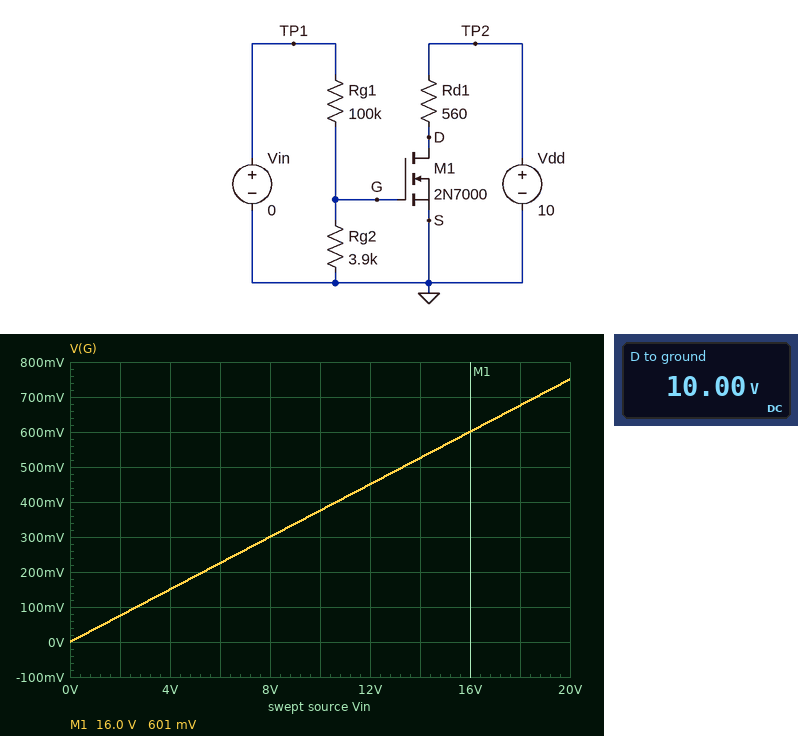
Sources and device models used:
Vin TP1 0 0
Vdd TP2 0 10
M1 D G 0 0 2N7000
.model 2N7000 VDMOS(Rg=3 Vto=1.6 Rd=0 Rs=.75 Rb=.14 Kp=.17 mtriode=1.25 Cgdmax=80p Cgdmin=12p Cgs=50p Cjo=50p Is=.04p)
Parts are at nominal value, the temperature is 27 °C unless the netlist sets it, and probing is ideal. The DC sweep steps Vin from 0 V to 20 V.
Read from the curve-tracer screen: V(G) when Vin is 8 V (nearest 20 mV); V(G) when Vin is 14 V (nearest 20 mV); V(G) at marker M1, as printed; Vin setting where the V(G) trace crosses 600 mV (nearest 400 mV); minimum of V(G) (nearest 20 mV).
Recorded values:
300 mV
520 mV
601 mV
16.0 V
0 V
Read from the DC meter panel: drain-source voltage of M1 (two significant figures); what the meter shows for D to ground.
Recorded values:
10 V
10.00 V
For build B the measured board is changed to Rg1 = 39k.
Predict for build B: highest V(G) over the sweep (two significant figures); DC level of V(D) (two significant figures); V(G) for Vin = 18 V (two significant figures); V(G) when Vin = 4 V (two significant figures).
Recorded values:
1.8 V
10 V
1.6 V
360 mV
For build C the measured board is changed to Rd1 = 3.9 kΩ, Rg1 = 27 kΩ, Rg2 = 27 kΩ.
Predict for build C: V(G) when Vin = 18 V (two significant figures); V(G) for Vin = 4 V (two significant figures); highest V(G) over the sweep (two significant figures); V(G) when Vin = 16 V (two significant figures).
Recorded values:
9.0 V
2.0 V
10 V
8.0 V
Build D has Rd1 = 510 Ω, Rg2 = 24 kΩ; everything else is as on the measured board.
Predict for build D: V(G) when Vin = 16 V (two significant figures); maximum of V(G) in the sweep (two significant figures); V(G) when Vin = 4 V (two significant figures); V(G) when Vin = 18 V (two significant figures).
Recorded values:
3.1 V
3.9 V
770 mV
3.5 V
